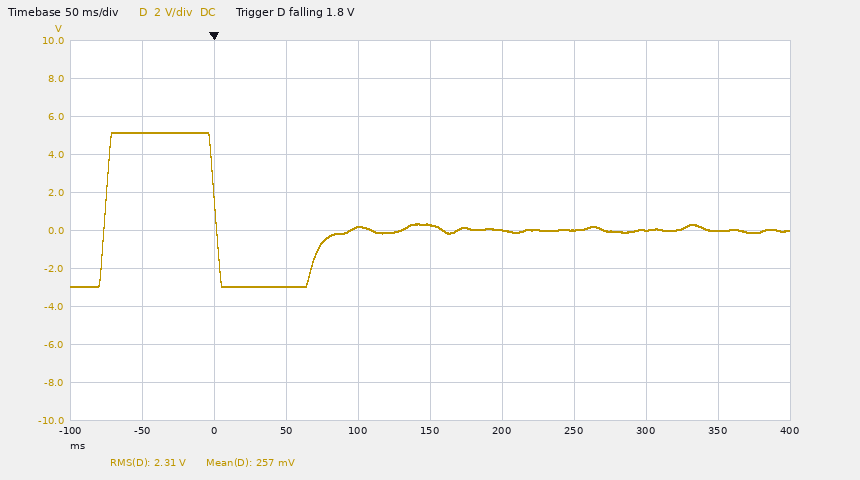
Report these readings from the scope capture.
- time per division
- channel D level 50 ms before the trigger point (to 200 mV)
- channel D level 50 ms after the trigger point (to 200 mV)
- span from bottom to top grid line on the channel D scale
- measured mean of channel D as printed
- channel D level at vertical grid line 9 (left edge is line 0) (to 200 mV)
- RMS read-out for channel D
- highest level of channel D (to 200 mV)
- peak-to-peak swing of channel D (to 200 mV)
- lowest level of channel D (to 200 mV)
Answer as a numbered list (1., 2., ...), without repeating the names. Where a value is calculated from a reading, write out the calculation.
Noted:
1. 50 ms
2. 5.2 V
3. -3.0 V
4. 20 V
5. 257 mV
6. 0.0 V
7. 2.31 V
8. 5.2 V
9. 5.2 V − (-3.0 V) = 8.2 V
10. -3.0 V
